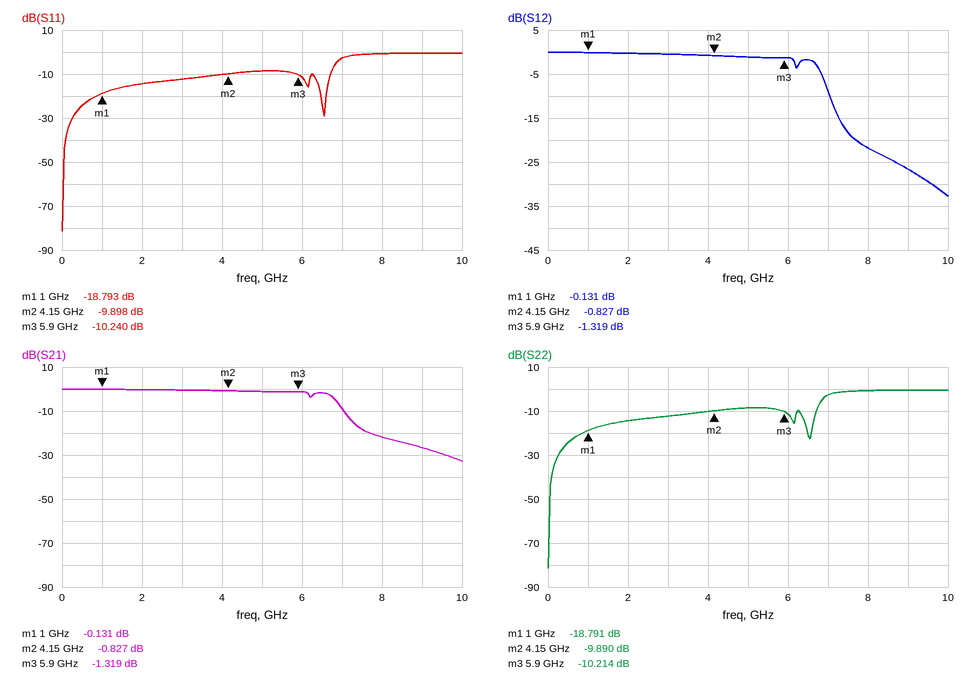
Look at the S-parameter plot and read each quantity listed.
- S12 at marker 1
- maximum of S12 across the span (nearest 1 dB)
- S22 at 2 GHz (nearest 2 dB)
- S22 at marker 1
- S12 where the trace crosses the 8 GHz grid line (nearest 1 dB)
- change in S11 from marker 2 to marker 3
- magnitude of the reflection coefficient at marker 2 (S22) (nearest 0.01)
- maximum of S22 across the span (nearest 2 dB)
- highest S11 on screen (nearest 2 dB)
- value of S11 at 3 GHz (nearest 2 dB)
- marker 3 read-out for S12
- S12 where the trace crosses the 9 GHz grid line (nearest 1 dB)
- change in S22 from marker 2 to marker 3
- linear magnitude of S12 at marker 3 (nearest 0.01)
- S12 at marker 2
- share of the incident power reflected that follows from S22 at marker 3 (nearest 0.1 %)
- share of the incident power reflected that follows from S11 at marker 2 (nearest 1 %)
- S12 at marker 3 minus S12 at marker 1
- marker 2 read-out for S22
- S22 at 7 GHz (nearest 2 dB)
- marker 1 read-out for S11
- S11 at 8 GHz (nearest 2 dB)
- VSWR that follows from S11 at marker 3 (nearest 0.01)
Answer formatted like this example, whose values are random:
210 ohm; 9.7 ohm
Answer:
-0.131 dB; 0 dB; -14 dB; -18.791 dB; -22 dB; -0.342 dB; 0.32; 0 dB; 0 dB; -12 dB; -1.319 dB; -27 dB; -0.324 dB; 0.86; -0.827 dB; 9.5 %; 10 %; -1.188 dB; -9.890 dB; -2 dB; -18.793 dB; 0 dB; 1.89
